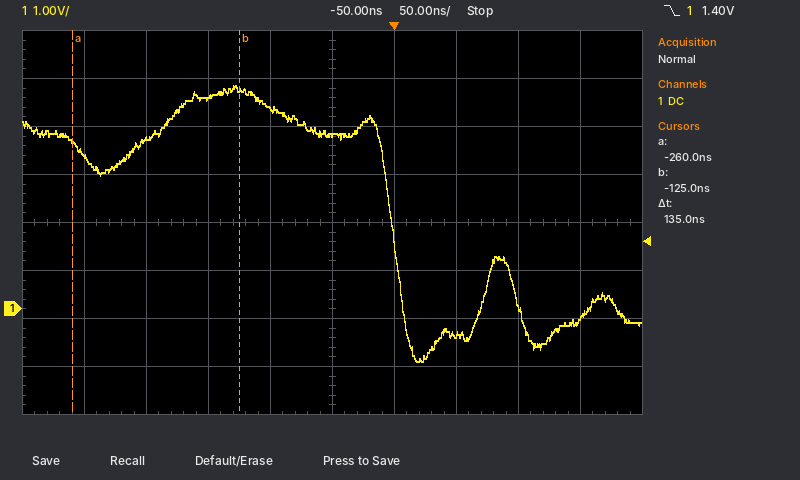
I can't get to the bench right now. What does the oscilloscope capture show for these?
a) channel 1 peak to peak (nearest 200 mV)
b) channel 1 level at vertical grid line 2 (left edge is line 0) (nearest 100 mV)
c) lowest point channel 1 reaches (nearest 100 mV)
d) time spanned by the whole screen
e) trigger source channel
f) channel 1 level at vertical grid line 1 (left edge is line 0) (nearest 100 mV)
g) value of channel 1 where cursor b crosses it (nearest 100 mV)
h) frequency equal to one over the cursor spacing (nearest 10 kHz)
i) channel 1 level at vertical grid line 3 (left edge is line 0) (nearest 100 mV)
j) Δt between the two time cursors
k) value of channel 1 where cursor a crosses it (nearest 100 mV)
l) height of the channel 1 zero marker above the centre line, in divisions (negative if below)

5.8 V
3.5 V
-1.1 V
500 ns
channel 1
3.2 V
4.6 V
7.41 MHz
4.4 V
135 ns
3.5 V
-1.8 div
